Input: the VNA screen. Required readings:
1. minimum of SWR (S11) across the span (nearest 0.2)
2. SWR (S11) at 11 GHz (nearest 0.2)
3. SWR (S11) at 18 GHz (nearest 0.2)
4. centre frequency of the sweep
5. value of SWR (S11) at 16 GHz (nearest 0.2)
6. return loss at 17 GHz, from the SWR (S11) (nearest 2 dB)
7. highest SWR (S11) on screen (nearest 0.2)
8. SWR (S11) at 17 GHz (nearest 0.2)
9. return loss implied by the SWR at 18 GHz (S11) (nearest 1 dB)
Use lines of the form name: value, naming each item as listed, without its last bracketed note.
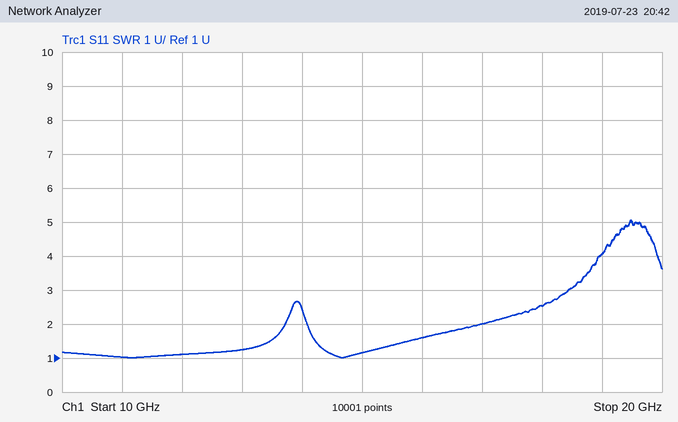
minimum of SWR (S11) across the span: 1.0
SWR (S11) at 11 GHz: 1.0
SWR (S11) at 18 GHz: 2.6
centre frequency of the sweep: 15 GHz
value of SWR (S11) at 16 GHz: 1.6
return loss at 17 GHz, from the SWR (S11): 10 dB
highest SWR (S11) on screen: 5.0
SWR (S11) at 17 GHz: 2.0
return loss implied by the SWR at 18 GHz (S11): 7 dB
